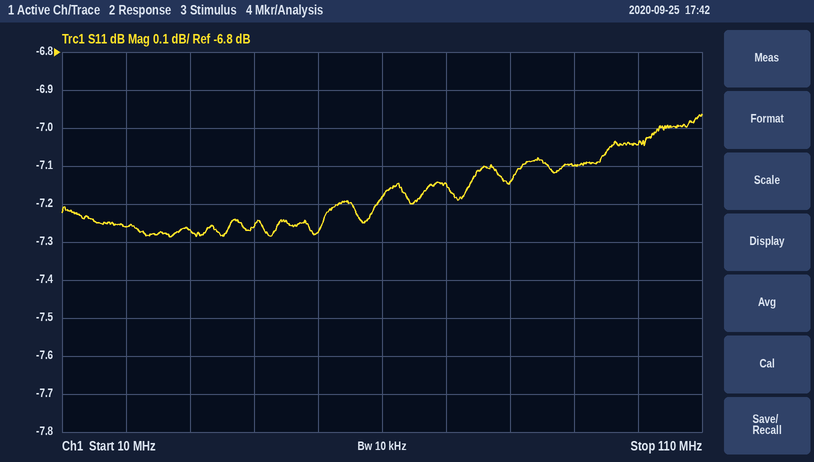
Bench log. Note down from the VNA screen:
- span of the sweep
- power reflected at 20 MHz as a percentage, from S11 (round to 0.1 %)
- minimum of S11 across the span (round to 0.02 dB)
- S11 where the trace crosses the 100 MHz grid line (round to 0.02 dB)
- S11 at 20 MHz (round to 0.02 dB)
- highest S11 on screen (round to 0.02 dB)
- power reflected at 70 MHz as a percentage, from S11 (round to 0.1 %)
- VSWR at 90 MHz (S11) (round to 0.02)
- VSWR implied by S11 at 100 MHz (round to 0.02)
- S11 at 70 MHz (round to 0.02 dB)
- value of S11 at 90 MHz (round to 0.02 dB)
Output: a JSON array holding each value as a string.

["100 MHz", "18.8 %", "-7.28 dB", "-7.04 dB", "-7.26 dB", "-6.96 dB", "19.3 %", "2.58", "2.60", "-7.14 dB", "-7.10 dB"]
